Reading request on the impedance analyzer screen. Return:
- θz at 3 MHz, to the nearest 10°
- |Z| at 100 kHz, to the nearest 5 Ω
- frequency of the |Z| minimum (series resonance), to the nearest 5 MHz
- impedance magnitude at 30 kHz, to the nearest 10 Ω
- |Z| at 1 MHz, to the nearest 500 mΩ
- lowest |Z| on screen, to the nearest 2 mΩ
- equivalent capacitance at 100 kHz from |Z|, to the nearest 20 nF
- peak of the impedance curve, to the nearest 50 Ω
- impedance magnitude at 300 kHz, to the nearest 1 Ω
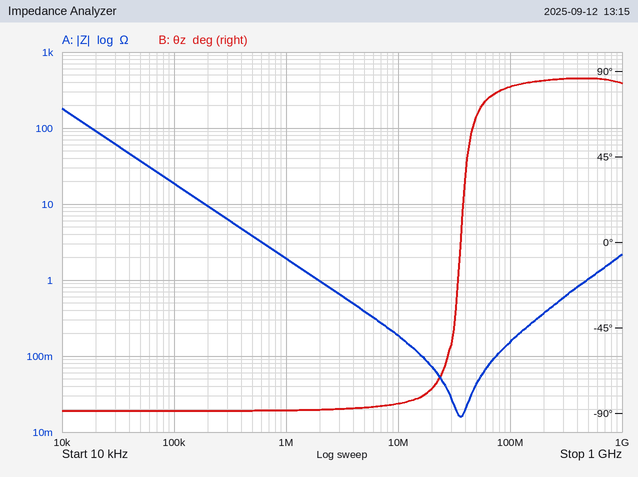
-90°
20 Ω
35 MHz
60 Ω
2.0 Ω
16 mΩ
80 nF
200 Ω
6 Ω
